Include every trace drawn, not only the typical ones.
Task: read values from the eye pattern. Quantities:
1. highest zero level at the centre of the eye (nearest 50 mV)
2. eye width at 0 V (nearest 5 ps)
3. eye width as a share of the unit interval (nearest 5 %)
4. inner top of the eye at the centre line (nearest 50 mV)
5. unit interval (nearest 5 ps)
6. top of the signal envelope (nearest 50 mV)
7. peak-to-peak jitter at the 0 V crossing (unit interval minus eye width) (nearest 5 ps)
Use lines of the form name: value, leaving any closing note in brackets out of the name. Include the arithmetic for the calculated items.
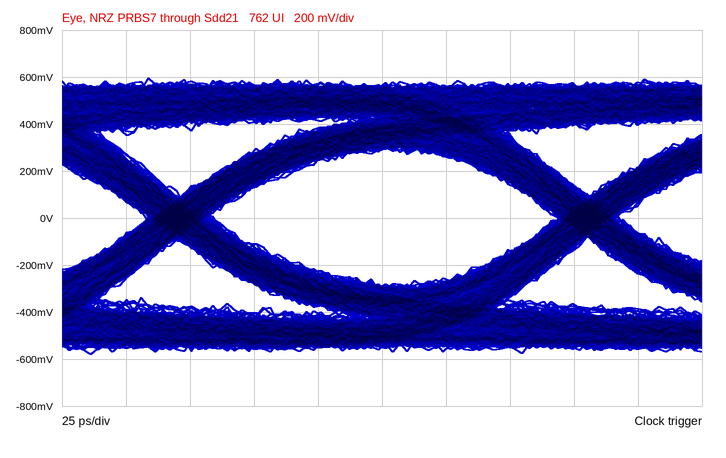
highest zero level at the centre of the eye: -300 mV
eye width at 0 V: 135 ps
eye width as a share of the unit interval: 135 ps / 160 ps ≈ 84.4 %, so 85 % to the nearest 5 %
inner top of the eye at the centre line: 300 mV
unit interval: 160 ps
top of the signal envelope: 600 mV
peak-to-peak jitter at the 0 V crossing (unit interval minus eye width): 25 ps
